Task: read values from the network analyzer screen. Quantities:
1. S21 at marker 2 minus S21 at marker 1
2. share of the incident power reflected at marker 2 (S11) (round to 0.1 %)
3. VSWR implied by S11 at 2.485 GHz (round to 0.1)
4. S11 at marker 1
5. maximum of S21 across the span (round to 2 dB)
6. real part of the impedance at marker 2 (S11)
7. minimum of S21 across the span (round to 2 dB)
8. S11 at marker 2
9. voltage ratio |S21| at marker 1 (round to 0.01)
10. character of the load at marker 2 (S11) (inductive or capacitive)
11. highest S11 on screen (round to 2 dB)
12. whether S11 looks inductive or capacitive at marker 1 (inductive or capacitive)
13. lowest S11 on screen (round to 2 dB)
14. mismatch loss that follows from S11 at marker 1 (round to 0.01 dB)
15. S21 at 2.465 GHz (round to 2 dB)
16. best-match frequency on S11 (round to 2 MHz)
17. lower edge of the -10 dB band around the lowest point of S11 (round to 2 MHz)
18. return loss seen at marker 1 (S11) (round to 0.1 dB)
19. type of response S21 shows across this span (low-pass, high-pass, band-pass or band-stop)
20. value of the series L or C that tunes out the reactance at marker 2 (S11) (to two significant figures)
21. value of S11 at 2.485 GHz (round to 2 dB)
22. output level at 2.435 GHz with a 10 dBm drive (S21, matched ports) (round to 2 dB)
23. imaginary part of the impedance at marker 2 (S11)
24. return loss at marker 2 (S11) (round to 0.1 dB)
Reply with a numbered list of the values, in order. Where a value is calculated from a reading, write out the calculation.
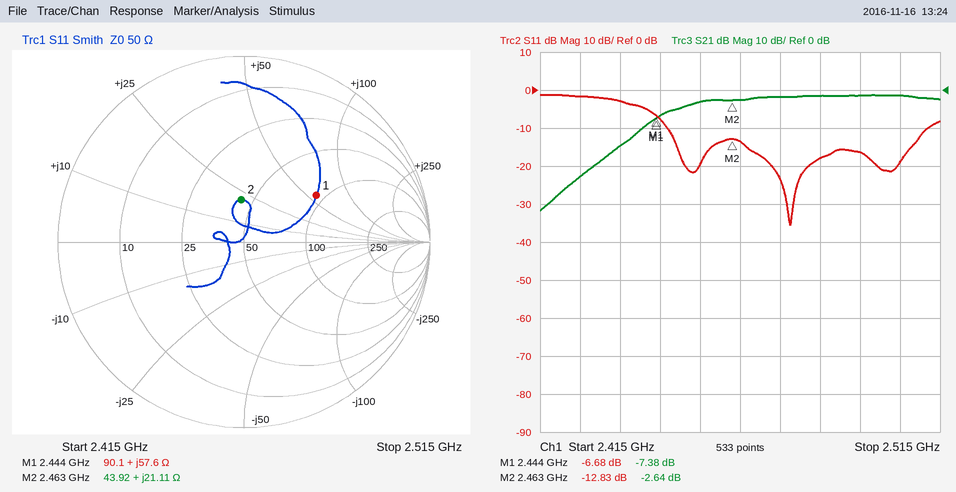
1. -2.64 − (-7.38) = 4.74 dB
2. 10^(-12.83/10) ≈ 5.2 %
3. |Γ| = 10^(-18/20) = 0.1259; VSWR = (1 + 0.1259)/(1 − 0.1259) ≈ 1.3
4. -6.68 dB
5. -2 dB
6. 43.92 Ω
7. -32 dB
8. -12.83 dB
9. 10^(-7.38/20) ≈ 0.43
10. inductive
11. -2 dB
12. inductive
13. -36 dB
14. −10 log10(1 − 10^(-6.68/10)) ≈ 1.05 dB
15. -2 dB
16. 2.478 GHz
17. 2.446 GHz
18. 6.7 dB
19. high-pass
20. C = 1/(2π × 2.463 GHz × 21.11 Ω) ≈ 3.1 pF
21. -18 dB
22. 10 dBm + (-14 dB) = -4 dBm
23. +21.11 Ω
24. 12.8 dB
